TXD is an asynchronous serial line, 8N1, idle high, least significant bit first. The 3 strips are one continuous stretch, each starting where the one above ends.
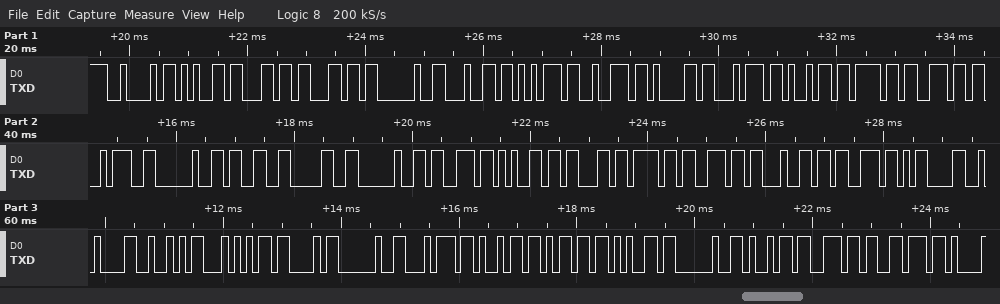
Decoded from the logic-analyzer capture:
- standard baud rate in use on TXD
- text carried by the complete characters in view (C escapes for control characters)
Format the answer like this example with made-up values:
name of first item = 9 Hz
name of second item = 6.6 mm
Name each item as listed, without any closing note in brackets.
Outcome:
standard baud rate in use on TXD = 9600 baud
text carried by the complete characters in view = "Bell duration: 30 seconds\r\nRTC time inv"
